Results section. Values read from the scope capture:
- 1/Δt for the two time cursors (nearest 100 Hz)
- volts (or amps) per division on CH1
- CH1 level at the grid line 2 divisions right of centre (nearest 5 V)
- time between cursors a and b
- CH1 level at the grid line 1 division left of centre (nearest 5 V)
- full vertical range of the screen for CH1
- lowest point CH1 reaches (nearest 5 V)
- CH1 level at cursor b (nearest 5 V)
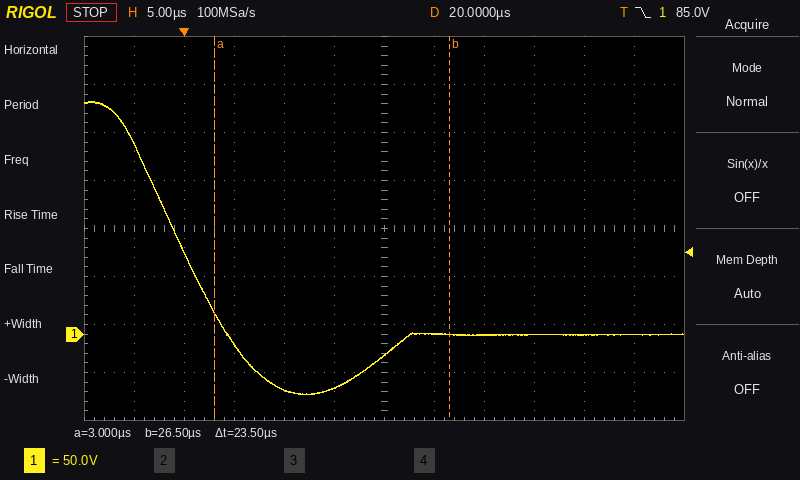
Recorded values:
42.6 kHz
50 V
0 V
23.5 µs
-55 V
400 V
-65 V
0 V
